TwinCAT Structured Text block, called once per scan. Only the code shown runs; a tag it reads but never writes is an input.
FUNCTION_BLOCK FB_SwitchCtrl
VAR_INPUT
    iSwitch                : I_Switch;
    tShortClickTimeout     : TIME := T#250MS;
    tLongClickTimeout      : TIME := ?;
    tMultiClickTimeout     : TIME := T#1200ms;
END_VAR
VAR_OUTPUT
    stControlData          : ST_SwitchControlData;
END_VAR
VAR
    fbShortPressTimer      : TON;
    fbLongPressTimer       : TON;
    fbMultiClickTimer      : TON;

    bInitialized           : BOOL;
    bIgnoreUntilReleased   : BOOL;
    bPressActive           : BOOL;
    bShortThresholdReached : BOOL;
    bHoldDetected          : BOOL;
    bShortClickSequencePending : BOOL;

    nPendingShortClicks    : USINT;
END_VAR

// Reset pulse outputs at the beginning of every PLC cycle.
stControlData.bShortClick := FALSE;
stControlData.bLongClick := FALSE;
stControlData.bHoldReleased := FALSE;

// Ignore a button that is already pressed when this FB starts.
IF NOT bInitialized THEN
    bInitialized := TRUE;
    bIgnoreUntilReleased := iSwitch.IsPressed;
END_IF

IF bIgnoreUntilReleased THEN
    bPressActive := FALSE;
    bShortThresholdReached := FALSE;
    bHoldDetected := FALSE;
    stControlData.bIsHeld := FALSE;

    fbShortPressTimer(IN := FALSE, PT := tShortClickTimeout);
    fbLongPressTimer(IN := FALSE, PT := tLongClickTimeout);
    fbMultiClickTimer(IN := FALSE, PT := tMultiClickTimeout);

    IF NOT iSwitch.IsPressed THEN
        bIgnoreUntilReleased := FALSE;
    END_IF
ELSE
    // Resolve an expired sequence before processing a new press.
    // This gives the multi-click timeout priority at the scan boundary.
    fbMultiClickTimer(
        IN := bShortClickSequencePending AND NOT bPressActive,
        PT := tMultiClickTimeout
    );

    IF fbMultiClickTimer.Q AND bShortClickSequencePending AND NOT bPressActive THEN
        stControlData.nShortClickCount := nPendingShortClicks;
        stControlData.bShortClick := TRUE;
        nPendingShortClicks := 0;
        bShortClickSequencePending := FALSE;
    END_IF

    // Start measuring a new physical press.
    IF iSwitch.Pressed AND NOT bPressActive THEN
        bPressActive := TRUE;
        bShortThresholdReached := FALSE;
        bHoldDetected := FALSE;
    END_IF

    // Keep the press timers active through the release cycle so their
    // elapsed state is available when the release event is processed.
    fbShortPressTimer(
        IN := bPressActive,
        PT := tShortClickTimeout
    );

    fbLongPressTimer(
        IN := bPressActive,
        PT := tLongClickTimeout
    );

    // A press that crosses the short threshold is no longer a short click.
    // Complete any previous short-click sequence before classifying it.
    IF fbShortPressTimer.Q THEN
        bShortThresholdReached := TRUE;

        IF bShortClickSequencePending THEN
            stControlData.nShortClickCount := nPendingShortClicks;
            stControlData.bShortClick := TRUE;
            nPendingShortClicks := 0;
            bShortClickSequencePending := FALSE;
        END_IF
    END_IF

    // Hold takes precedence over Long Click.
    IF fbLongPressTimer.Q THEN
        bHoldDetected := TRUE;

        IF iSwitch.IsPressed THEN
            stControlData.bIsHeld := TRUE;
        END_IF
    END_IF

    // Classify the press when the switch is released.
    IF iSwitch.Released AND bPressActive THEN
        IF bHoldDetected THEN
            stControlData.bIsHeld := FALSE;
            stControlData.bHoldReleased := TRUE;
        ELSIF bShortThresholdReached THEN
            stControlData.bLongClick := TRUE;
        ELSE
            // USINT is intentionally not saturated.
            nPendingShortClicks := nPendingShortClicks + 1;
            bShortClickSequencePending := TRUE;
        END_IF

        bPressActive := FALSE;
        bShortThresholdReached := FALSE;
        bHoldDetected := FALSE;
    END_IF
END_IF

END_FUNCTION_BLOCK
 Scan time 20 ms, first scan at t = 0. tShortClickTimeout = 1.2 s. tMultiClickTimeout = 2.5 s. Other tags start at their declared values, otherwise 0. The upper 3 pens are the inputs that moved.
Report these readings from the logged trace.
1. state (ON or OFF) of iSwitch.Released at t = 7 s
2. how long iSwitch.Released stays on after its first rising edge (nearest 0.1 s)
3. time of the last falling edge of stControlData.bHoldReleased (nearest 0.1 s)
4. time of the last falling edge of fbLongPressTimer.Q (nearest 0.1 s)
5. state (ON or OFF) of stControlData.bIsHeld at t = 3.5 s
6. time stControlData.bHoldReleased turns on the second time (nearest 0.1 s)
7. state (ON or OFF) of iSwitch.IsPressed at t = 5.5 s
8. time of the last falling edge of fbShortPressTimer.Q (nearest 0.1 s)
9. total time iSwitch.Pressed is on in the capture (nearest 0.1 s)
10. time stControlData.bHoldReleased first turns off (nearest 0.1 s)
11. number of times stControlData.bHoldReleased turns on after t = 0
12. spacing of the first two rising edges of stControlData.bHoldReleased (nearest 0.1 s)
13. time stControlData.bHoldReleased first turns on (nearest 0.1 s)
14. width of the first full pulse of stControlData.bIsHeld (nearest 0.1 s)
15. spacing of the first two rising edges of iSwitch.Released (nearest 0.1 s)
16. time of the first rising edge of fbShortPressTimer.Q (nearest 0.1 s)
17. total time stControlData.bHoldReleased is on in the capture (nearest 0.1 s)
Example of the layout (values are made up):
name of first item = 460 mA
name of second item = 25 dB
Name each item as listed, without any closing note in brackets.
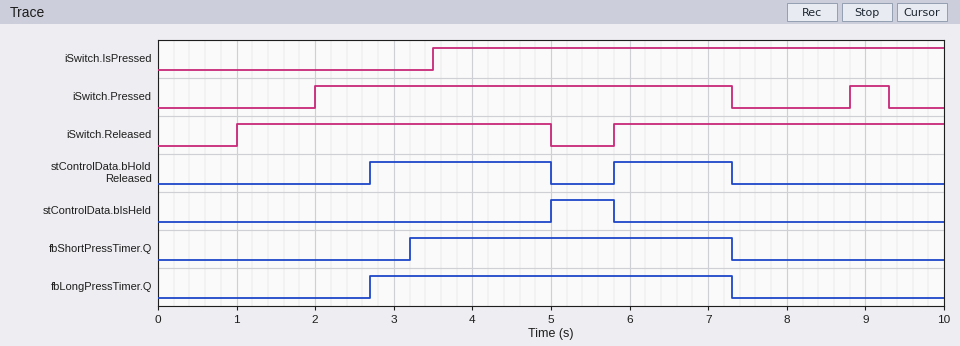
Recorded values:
state (ON or OFF) of iSwitch.Released at t = 7 s = ON
how long iSwitch.Released stays on after its first rising edge = 4.0 s
time of the last falling edge of stControlData.bHoldReleased = 7.3 s
time of the last falling edge of fbLongPressTimer.Q = 7.3 s
state (ON or OFF) of stControlData.bIsHeld at t = 3.5 s = OFF
time stControlData.bHoldReleased turns on the second time = 5.8 s
state (ON or OFF) of iSwitch.IsPressed at t = 5.5 s = ON
time of the last falling edge of fbShortPressTimer.Q = 7.3 s
total time iSwitch.Pressed is on in the capture = 5.8 s
time stControlData.bHoldReleased first turns off = 5.0 s
number of times stControlData.bHoldReleased turns on after t = 0 = 2
spacing of the first two rising edges of stControlData.bHoldReleased = 3.1 s
time stControlData.bHoldReleased first turns on = 2.7 s
width of the first full pulse of stControlData.bIsHeld = 0.8 s
spacing of the first two rising edges of iSwitch.Released = 4.8 s
time of the first rising edge of fbShortPressTimer.Q = 3.2 s
total time stControlData.bHoldReleased is on in the capture = 3.8 s
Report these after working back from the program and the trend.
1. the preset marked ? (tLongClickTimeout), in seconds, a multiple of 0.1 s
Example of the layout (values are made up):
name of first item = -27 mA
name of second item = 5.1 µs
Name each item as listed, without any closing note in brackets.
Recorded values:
the preset marked ? (tLongClickTimeout), in seconds, a multiple of 0.1 s = 0.7 s
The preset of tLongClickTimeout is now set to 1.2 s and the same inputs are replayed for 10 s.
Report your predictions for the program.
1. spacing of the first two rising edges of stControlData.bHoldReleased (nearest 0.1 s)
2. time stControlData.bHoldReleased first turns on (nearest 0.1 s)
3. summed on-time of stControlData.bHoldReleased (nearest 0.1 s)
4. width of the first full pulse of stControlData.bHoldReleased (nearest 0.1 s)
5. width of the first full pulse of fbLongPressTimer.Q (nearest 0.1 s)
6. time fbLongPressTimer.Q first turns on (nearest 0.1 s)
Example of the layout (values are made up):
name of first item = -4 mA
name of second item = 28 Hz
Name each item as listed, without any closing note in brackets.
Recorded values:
spacing of the first two rising edges of stControlData.bHoldReleased = 2.6 s
time stControlData.bHoldReleased first turns on = 3.2 s
summed on-time of stControlData.bHoldReleased = 3.3 s
width of the first full pulse of stControlData.bHoldReleased = 1.8 s
width of the first full pulse of fbLongPressTimer.Q = 4.1 s
time fbLongPressTimer.Q first turns on = 3.2 s
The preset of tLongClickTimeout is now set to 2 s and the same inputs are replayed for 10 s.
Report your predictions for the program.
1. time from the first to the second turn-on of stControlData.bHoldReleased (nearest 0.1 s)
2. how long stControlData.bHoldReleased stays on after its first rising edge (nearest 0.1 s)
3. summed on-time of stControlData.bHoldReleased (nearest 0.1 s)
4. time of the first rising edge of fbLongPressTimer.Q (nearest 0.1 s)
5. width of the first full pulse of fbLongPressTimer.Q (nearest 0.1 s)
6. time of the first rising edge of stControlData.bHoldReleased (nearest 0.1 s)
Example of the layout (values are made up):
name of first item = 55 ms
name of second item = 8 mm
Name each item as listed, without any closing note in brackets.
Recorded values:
time from the first to the second turn-on of stControlData.bHoldReleased = 1.8 s
how long stControlData.bHoldReleased stays on after its first rising edge = 1.0 s
summed on-time of stControlData.bHoldReleased = 2.5 s
time of the first rising edge of fbLongPressTimer.Q = 4.0 s
width of the first full pulse of fbLongPressTimer.Q = 3.3 s
time of the first rising edge of stControlData.bHoldReleased = 4.0 s
